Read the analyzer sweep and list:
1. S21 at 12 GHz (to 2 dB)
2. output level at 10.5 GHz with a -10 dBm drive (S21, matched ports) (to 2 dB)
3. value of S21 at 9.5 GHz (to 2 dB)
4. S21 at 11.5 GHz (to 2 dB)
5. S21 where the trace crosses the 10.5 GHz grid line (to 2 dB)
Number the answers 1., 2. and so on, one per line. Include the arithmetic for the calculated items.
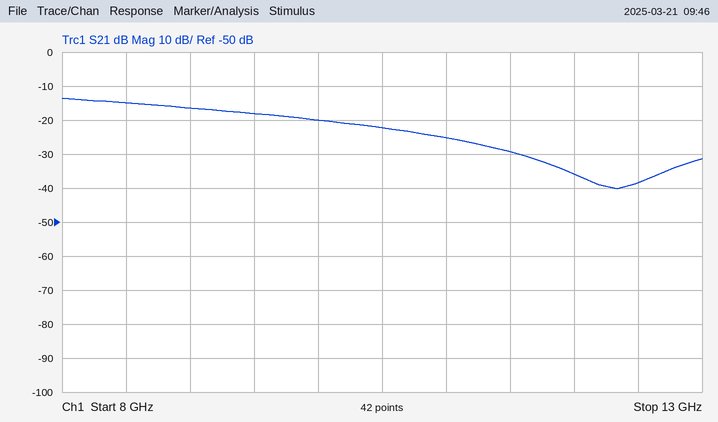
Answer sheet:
1. -36 dB
2. -10 dBm + (-22 dB) = -32 dBm
3. -18 dB
4. -30 dB
5. -22 dB
